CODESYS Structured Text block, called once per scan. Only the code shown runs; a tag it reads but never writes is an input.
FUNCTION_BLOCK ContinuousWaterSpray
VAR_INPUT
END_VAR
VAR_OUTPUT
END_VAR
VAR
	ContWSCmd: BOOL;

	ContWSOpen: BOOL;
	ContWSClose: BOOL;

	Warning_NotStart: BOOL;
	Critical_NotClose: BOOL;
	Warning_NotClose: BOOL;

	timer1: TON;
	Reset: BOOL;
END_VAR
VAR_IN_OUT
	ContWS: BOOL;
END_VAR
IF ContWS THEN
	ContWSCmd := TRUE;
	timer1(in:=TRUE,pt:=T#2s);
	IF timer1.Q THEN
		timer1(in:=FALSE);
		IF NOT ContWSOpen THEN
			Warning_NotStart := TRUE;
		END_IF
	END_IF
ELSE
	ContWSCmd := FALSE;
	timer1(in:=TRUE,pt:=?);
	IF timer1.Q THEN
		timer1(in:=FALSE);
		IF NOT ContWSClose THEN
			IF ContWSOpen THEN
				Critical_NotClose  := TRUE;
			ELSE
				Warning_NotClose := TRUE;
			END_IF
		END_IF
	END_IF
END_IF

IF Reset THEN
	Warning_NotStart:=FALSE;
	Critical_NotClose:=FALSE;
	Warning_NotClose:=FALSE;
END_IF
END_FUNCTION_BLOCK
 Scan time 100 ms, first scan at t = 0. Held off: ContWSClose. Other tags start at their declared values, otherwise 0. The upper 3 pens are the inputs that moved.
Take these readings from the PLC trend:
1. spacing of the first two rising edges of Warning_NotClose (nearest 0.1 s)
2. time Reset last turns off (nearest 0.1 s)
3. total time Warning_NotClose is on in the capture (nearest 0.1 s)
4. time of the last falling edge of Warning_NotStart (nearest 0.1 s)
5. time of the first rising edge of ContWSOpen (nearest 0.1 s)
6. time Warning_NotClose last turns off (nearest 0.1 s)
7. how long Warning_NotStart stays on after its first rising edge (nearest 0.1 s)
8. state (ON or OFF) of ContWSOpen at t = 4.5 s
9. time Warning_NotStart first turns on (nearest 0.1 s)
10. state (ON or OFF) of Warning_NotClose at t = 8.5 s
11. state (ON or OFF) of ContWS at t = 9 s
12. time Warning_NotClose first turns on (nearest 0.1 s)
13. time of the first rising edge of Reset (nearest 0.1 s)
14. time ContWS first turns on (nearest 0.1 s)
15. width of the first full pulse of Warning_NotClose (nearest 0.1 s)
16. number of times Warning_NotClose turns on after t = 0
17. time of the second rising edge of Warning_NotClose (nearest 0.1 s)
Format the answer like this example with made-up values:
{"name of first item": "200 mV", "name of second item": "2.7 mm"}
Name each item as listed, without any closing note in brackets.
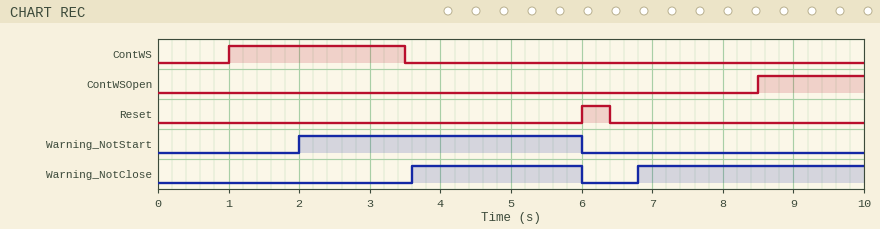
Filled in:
{"spacing of the first two rising edges of Warning_NotClose": "3.2 s", "time Reset last turns off": "6.4 s", "total time Warning_NotClose is on in the capture": "5.6 s", "time of the last falling edge of Warning_NotStart": "6.0 s", "time of the first rising edge of ContWSOpen": "8.5 s", "time Warning_NotClose last turns off": "6.0 s", "how long Warning_NotStart stays on after its first rising edge": "4.0 s", "state (ON or OFF) of ContWSOpen at t = 4.5 s": "OFF", "time Warning_NotStart first turns on": "2.0 s", "state (ON or OFF) of Warning_NotClose at t = 8.5 s": "ON", "state (ON or OFF) of ContWS at t = 9 s": "OFF", "time Warning_NotClose first turns on": "3.6 s", "time of the first rising edge of Reset": "6.0 s", "time ContWS first turns on": "1.0 s", "width of the first full pulse of Warning_NotClose": "2.4 s", "number of times Warning_NotClose turns on after t = 0": "2", "time of the second rising edge of Warning_NotClose": "6.8 s"}
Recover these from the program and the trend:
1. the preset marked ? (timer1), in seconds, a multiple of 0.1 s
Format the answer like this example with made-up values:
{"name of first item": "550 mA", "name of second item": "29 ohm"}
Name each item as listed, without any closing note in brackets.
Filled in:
{"the preset marked ? (timer1), in seconds, a multiple of 0.1 s": "1.5 s"}
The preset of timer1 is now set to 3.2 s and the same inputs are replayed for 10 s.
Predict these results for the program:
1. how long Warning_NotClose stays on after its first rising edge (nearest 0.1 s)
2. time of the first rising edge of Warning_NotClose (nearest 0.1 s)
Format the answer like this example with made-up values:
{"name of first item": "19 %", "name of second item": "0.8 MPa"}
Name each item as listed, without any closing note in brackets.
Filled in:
{"how long Warning_NotClose stays on after its first rising edge": "0.7 s", "time of the first rising edge of Warning_NotClose": "5.3 s"}
